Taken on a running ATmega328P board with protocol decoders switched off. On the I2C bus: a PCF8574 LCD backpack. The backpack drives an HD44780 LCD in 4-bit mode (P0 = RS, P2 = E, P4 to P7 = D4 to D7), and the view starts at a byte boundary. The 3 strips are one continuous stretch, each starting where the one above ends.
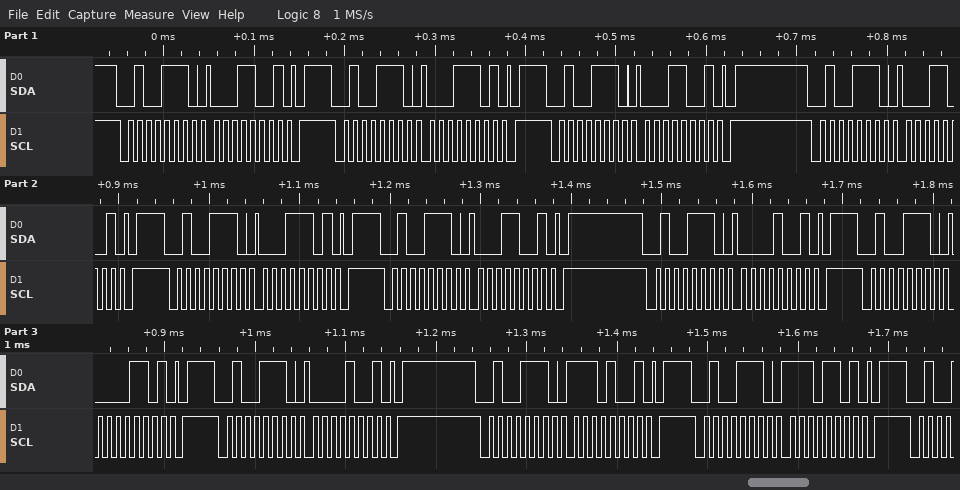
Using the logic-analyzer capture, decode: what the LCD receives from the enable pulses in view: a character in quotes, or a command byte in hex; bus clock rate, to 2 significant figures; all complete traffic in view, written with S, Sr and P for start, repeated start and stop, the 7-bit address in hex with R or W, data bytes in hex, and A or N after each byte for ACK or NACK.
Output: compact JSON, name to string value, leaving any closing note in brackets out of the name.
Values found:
{"what the LCD receives from the enable pulses in view: a character in quotes, or a command byte in hex": "data 0x11", "bus clock rate, to 2 significant figures": "100 kHz", "all complete traffic in view, written with S, Sr and P for start, repeated start and stop, the 7-bit address in hex with R or W, data bytes in hex, and A or N after each byte for ACK or NACK": "S 27W A 19 A P S 27W A 1D A P S 27W A 19 A P S 27W A 19 A P S 27W A 1D A P S 27W A 19 A P S 27W A 09 A P S 27W A 0D A P S 27W A 09 A P S 27W A E9 A P S 27W A ED A P"}
